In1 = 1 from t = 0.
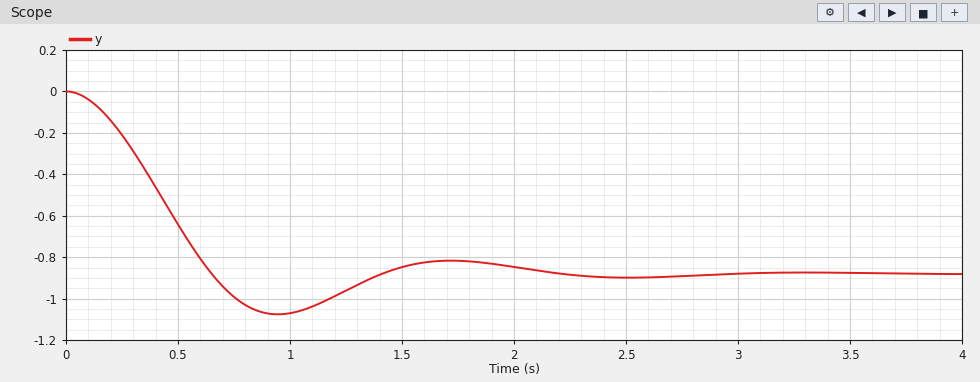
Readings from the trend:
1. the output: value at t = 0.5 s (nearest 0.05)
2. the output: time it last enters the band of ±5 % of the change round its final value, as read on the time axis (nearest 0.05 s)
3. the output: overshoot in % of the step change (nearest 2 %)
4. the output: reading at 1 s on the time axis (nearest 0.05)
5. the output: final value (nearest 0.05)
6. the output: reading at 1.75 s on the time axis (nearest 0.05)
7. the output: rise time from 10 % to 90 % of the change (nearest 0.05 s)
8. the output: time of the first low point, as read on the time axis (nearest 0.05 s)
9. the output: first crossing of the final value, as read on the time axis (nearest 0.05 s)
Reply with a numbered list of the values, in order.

1. -0.65
2. 1.95 s
3. 22 %
4. -1.05
5. -0.90
6. -0.80
7. 0.45 s
8. 0.95 s
9. 0.65 s
